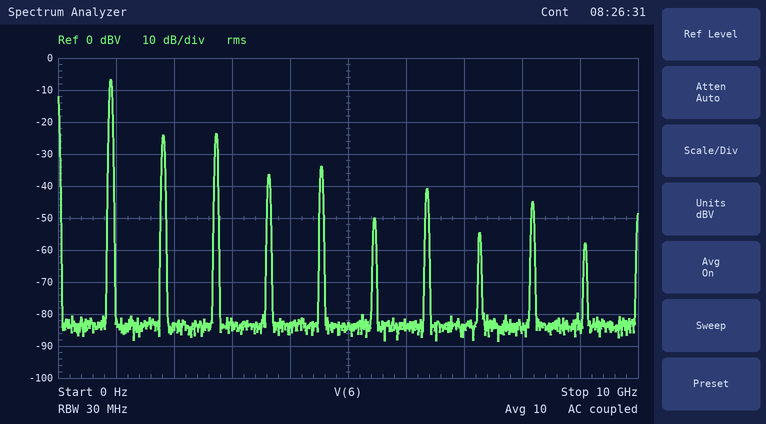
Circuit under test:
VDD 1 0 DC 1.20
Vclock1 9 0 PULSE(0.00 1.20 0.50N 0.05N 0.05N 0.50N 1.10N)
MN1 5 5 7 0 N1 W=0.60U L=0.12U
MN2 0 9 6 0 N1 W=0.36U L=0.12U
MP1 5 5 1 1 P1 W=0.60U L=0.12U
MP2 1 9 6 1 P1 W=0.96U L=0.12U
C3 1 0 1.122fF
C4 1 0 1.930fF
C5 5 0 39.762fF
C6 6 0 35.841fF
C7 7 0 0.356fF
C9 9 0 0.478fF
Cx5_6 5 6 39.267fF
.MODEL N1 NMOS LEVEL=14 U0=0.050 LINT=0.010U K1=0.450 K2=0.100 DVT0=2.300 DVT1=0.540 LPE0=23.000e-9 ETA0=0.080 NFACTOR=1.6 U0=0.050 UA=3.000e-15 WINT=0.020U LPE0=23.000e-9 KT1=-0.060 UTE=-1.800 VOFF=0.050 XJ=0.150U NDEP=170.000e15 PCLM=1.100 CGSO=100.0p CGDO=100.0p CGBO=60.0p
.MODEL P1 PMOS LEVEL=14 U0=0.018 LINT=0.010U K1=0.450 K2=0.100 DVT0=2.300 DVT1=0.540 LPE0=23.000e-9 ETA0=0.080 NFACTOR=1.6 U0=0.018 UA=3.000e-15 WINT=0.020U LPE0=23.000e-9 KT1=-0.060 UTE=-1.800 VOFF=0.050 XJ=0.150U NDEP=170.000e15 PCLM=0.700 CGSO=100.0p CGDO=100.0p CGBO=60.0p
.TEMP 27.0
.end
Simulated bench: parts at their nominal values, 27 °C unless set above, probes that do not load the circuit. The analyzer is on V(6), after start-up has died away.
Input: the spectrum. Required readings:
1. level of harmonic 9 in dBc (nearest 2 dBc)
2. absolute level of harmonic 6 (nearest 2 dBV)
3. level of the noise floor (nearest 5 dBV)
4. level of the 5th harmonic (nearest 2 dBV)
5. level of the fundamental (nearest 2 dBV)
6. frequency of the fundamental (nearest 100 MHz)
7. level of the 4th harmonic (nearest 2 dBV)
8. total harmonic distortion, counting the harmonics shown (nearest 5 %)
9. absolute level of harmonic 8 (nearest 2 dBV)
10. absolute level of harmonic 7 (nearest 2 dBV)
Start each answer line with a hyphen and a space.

- -38 dBc
- -50 dBV
- -85 dBV
- -34 dBV
- -6 dBV
- 900 MHz
- -36 dBV
- 20 %
- -54 dBV
- -40 dBV
